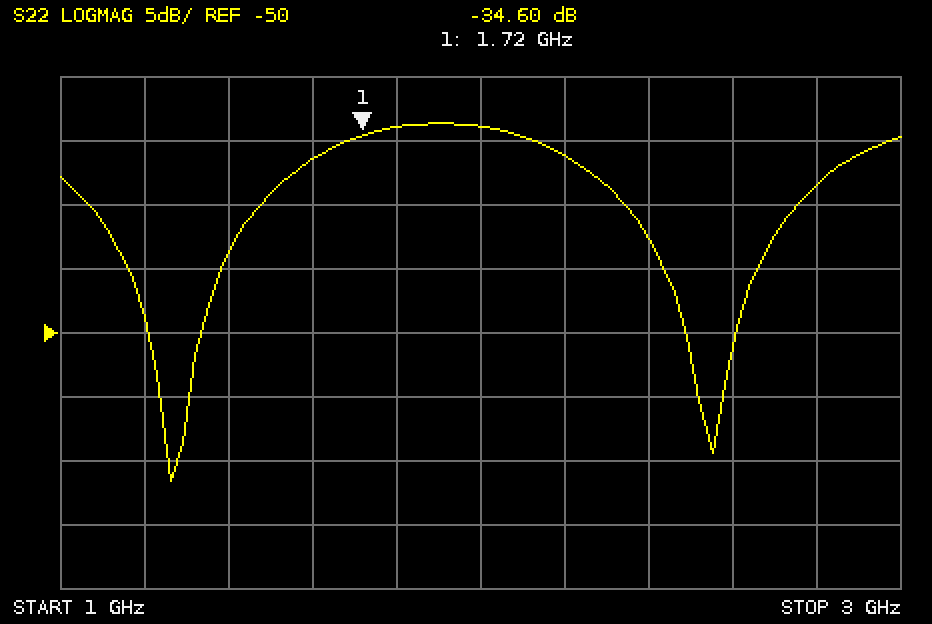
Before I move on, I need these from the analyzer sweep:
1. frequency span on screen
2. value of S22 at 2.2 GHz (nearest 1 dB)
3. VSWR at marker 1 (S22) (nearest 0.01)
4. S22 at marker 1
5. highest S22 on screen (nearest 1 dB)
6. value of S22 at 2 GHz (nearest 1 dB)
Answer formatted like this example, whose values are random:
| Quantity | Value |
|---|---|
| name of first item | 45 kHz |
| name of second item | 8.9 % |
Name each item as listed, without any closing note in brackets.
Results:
| Quantity | Value |
|---|---|
| frequency span on screen | 2 GHz |
| value of S22 at 2.2 GHz | -36 dB |
| VSWR at marker 1 (S22) | 1.04 |
| S22 at marker 1 | -34.60 dB |
| highest S22 on screen | -34 dB |
| value of S22 at 2 GHz | -34 dB |
